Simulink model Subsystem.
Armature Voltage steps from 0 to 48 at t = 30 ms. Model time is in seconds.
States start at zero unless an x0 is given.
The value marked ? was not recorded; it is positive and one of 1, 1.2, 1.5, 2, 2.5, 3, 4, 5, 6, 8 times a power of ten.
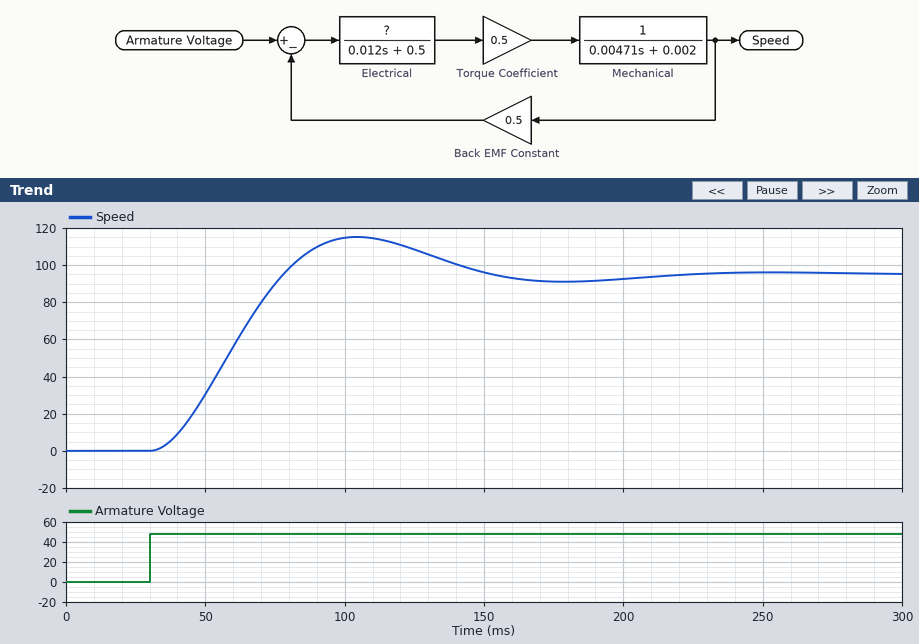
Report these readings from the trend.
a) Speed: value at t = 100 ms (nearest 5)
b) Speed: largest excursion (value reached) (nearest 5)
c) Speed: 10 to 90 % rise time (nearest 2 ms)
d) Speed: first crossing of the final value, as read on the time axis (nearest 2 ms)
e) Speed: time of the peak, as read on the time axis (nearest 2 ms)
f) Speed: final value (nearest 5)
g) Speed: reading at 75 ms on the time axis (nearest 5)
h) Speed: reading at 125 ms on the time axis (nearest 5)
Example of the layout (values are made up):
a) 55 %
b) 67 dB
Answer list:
a) 115
b) 115
c) 32 ms
d) 78 ms
e) 104 ms
f) 95
g) 90
h) 110
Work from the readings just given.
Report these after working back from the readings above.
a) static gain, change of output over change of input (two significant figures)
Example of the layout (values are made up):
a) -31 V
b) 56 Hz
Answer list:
a) 2.0
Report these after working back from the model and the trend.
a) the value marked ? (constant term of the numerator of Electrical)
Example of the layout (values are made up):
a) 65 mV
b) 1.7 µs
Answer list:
a) 0.5
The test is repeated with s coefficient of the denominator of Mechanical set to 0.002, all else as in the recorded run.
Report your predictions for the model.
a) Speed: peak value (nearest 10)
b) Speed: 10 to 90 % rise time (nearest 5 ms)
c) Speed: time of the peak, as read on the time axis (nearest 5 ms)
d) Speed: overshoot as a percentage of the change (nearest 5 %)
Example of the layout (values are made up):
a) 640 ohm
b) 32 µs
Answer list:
a) 130
b) 20 ms
c) 75 ms
d) 40 %
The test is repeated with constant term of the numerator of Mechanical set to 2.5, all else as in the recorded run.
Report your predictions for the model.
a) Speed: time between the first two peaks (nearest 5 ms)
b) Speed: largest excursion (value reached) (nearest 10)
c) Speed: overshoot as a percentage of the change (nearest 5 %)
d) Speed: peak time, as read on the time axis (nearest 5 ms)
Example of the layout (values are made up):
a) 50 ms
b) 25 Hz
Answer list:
a) 90 ms
b) 130
c) 40 %
d) 75 ms
